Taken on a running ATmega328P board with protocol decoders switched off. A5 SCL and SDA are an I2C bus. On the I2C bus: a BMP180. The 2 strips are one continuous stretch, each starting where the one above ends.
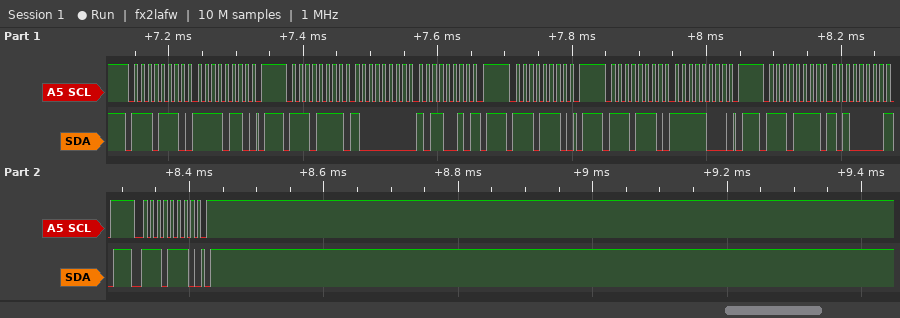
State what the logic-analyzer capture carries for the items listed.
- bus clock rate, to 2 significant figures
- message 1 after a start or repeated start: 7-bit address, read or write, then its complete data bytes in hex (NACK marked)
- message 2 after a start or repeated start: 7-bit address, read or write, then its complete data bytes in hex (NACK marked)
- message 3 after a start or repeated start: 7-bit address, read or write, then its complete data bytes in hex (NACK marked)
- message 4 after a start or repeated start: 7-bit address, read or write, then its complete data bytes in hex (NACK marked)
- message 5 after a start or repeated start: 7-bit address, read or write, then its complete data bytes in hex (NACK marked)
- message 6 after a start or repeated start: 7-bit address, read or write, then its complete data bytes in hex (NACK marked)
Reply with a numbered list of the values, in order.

1. 100 kHz
2. 0x77 write: F6
3. 0x77 read: 80 B2 NACK
4. 0x77 write
5. 0x77 write: F8
6. 0x77 read: A0 NACK
7. 0x77 write
